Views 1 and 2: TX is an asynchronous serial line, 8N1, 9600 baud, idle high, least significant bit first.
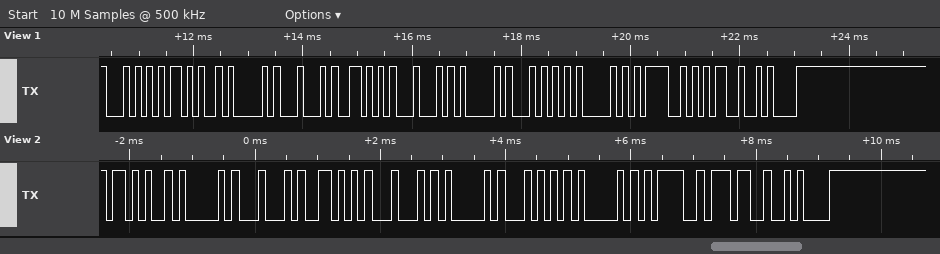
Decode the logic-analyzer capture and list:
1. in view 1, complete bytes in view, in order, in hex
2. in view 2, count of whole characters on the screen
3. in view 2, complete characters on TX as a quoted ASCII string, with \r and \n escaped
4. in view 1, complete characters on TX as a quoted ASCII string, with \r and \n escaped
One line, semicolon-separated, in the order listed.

0x54 0x2B 0x41 0x44 0x56 0x44 0x41 0x54 0x41 0x3D 0x35 0x0A; 11; "+ADVDATA=7\n"; "T+ADVDATA=5\n"
